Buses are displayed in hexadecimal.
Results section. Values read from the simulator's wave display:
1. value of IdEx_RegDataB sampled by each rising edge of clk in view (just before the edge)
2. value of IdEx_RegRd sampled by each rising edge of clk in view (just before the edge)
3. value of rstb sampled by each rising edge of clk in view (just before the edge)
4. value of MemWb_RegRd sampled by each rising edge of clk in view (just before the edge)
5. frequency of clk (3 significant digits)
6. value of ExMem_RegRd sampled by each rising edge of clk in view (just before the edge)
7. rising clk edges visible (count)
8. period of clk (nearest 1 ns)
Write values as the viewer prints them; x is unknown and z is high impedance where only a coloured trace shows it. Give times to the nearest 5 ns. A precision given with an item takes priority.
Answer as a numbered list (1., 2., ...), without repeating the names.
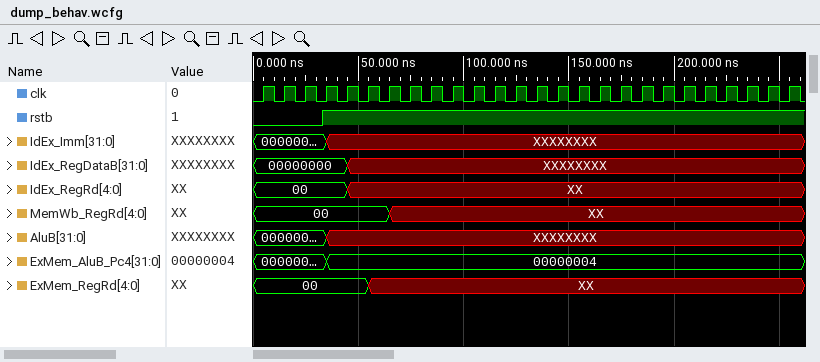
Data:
1. 00000000, 00000000, 00000000, 00000000, 00000000, XXXXXXXX, XXXXXXXX, XXXXXXXX, XXXXXXXX, XXXXXXXX, XXXXXXXX, XXXXXXXX, XXXXXXXX, XXXXXXXX, XXXXXXXX, XXXXXXXX, XXXXXXXX, XXXXXXXX, XXXXXXXX, XXXXXXXX, XXXXXXXX, XXXXXXXX, XXXXXXXX, XXXXXXXX, XXXXXXXX, XXXXXXXX
2. 00, 00, 00, 00, 00, XX, XX, XX, XX, XX, XX, XX, XX, XX, XX, XX, XX, XX, XX, XX, XX, XX, XX, XX, XX, XX
3. 0 0 0 1 1 1 1 1 1 1 1 1 1 1 1 1 1 1 1 1 1 1 1 1 1 1
4. 00, 00, 00, 00, 00, 00, 00, XX, XX, XX, XX, XX, XX, XX, XX, XX, XX, XX, XX, XX, XX, XX, XX, XX, XX, XX
5. 100 MHz
6. 00, 00, 00, 00, 00, 00, XX, XX, XX, XX, XX, XX, XX, XX, XX, XX, XX, XX, XX, XX, XX, XX, XX, XX, XX, XX
7. 26
8. 10 ns
